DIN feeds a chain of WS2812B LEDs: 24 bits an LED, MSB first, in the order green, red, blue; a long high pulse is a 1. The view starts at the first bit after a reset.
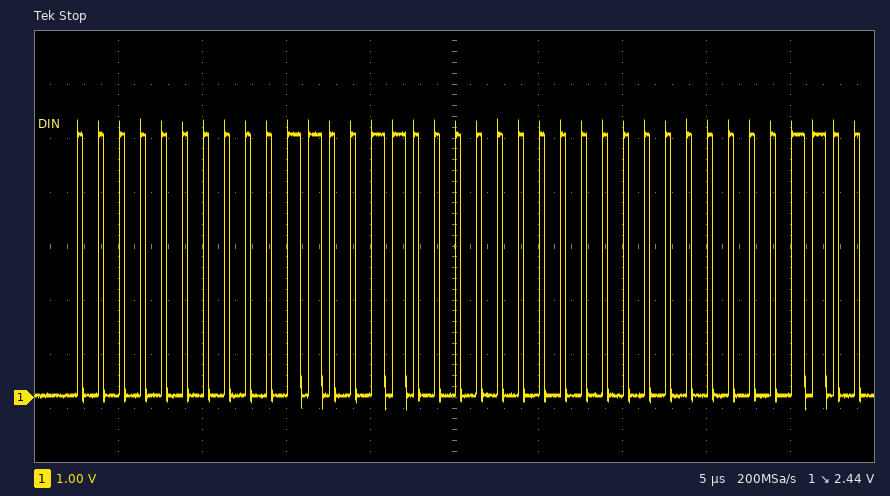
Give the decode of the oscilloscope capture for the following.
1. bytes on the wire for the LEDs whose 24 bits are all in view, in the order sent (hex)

00 33 00
